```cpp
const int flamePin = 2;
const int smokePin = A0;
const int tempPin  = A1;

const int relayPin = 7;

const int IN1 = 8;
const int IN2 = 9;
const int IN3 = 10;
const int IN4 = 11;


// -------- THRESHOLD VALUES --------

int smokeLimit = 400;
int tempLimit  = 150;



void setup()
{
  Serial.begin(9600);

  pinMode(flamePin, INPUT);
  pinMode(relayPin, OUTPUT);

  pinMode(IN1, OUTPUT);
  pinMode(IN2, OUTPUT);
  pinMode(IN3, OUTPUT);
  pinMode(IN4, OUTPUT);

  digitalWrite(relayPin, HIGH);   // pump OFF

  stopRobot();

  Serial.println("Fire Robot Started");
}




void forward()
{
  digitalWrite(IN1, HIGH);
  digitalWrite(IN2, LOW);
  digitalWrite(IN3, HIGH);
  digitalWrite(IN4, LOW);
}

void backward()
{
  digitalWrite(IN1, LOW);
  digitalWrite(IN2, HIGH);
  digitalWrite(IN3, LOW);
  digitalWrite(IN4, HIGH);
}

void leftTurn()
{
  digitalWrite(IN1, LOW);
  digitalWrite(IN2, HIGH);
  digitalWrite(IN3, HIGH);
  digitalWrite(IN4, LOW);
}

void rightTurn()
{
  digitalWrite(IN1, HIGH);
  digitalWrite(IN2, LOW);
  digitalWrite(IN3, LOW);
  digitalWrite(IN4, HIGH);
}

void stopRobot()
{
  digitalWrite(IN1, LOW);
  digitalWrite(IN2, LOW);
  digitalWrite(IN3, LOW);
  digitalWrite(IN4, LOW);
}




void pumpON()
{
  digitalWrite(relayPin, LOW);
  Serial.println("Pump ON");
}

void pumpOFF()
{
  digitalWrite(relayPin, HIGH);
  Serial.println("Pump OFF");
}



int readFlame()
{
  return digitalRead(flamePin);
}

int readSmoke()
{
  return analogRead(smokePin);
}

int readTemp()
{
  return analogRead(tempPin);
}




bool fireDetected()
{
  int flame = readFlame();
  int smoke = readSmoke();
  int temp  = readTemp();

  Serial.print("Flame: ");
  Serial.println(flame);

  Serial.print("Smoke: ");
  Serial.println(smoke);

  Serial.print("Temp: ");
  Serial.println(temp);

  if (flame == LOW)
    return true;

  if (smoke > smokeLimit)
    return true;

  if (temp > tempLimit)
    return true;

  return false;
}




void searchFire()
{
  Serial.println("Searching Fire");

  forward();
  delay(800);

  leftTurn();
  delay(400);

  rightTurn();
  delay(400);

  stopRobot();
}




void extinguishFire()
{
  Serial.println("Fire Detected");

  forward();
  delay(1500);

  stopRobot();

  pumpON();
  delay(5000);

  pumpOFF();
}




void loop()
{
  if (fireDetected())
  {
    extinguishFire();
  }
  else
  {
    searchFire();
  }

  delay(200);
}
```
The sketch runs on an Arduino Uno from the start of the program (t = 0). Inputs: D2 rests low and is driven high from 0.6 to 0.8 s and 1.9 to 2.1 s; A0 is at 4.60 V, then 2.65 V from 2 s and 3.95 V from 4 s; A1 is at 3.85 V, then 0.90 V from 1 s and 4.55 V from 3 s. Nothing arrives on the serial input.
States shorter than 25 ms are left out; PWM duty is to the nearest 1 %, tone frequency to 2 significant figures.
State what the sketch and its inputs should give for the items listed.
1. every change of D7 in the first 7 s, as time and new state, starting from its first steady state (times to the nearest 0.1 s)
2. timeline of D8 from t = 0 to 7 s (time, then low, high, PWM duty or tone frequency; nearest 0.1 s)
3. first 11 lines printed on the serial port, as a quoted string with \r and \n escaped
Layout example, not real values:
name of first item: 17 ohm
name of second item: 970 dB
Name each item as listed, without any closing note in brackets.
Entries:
every change of D7 in the first 7 s, as time and new state, starting from its first steady state: 0 s high; 1.5 s low; 6.5 s high
timeline of D8 from t = 0 to 7 s: 0 s high; 1.5 s low; 6.7 s high
first 11 lines printed on the serial port, as a quoted string with \r and \n escaped: "Fire Robot Started\r\nFlame: 0\r\nSmoke: 942\r\nTemp: 788\r\nFire Detected\r\nPump ON\r\nPump OFF\r\nFlame: 0\r\nSmoke: 808\r\nTemp: 931\r\nFire Detected\r\n"
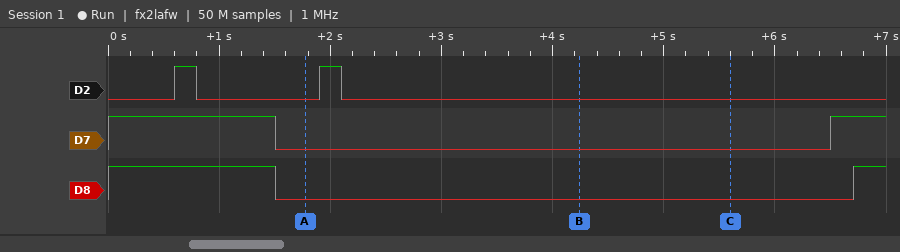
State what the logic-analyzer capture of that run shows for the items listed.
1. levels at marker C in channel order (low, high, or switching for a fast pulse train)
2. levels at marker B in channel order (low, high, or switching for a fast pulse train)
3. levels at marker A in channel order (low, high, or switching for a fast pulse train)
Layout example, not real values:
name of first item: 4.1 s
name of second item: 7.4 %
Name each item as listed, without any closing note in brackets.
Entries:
levels at marker C in channel order: D2 low, D7 low, D8 low
levels at marker B in channel order: D2 low, D7 low, D8 low
levels at marker A in channel order: D2 low, D7 low, D8 low
